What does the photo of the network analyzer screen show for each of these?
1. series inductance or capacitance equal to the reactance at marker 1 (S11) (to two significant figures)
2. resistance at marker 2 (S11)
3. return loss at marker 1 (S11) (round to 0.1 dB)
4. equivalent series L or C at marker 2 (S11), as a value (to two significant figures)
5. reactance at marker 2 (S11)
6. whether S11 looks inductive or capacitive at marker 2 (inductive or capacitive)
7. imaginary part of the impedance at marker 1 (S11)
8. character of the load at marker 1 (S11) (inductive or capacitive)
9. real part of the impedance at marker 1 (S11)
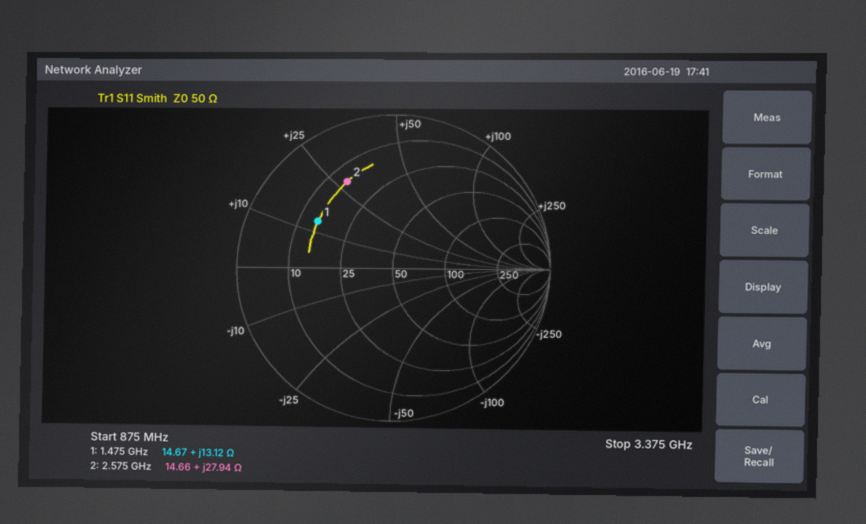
1.4 nH
14.66 Ω
4.9 dB
1.7 nH
+27.94 Ω
inductive
+13.12 Ω
inductive
14.67 Ω
